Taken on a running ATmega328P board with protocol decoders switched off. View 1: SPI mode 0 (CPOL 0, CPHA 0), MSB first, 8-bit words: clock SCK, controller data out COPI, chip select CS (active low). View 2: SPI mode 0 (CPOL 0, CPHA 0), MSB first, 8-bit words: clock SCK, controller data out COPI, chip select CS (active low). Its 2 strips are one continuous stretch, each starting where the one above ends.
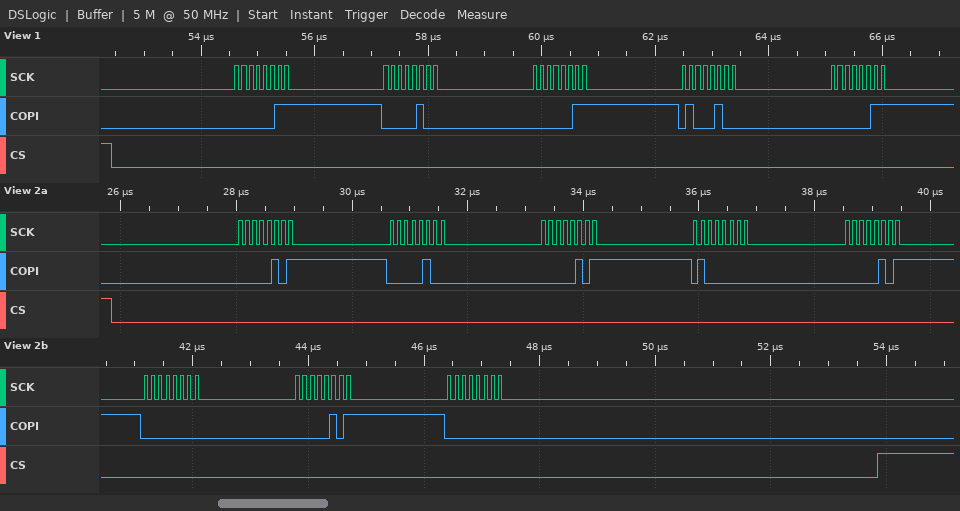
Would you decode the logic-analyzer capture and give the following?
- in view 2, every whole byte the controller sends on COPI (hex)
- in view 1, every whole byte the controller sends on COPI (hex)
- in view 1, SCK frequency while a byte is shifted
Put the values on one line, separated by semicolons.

05 04 05 40 05 00 05 00; 0x03 0x04 0x03 0x44 0x03; 8 MHz
